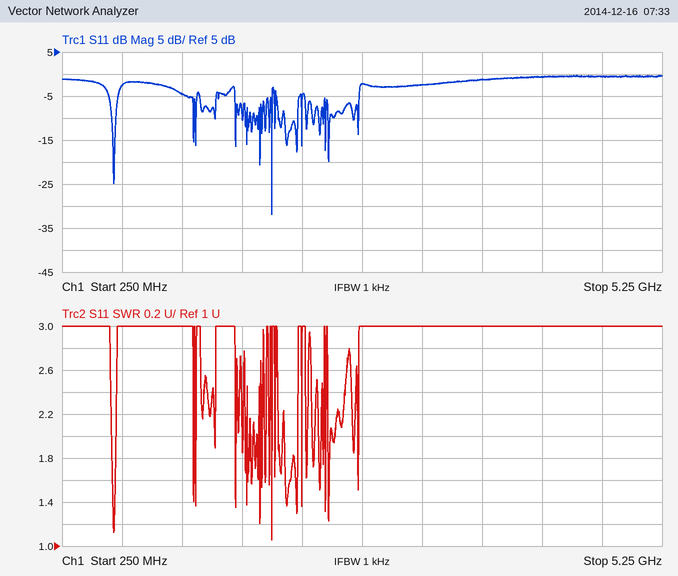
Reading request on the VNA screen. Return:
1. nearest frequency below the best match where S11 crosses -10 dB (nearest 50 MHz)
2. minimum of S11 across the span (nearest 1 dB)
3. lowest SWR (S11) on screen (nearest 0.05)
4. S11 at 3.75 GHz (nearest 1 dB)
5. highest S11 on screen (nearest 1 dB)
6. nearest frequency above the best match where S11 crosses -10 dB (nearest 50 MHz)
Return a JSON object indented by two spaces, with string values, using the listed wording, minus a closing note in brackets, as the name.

{
  "nearest frequency below the best match where S11 crosses -10 dB": "2.00 GHz",
  "minimum of S11 across the span": "-32 dB",
  "lowest SWR (S11) on screen": "1.05",
  "S11 at 3.75 GHz": "-1 dB",
  "highest S11 on screen": "0 dB",
  "nearest frequency above the best match where S11 crosses -10 dB": "2.00 GHz"
}
